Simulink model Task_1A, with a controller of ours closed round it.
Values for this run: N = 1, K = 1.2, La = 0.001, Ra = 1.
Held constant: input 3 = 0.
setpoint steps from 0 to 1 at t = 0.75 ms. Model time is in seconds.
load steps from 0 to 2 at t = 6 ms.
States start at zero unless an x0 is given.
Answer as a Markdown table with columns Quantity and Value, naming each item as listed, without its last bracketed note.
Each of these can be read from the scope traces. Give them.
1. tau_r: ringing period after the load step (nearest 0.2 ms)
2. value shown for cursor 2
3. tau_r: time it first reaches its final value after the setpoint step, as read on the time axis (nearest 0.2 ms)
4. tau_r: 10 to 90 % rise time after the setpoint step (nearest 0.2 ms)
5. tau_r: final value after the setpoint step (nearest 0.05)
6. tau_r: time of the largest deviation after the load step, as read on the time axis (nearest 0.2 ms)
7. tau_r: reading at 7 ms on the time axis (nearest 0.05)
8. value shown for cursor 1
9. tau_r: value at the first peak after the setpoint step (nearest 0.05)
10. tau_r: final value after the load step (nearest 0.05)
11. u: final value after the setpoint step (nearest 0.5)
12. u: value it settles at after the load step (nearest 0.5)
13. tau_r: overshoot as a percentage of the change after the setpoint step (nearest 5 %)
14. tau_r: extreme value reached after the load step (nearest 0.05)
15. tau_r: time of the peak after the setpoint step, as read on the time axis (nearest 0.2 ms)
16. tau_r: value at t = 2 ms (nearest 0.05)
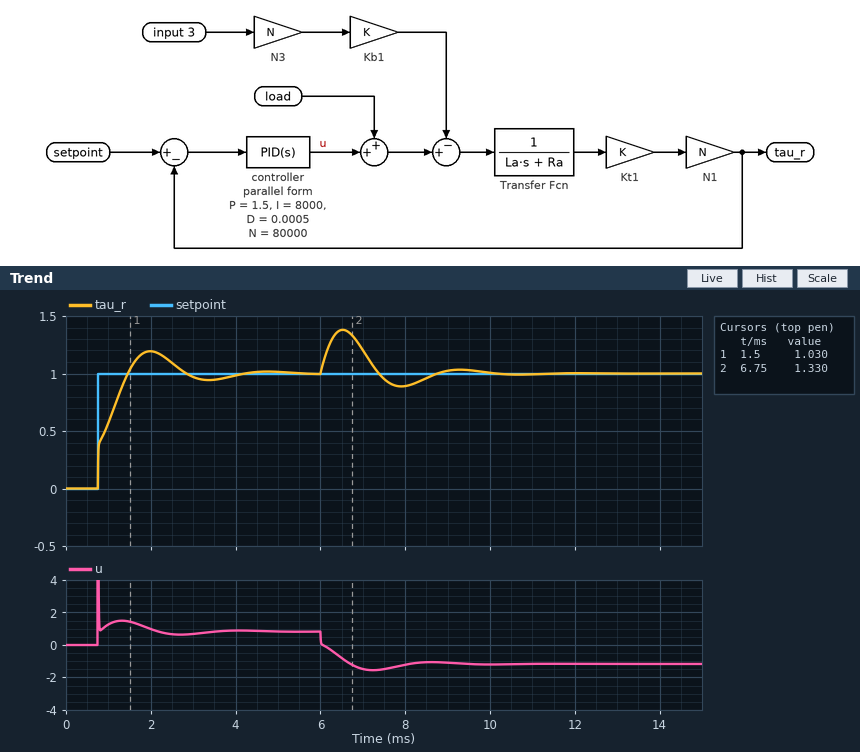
| Quantity | Value |
|---|---|
| tau_r: ringing period after the load step | 2.8 ms |
| value shown for cursor 2 | 1.330 |
| tau_r: time it first reaches its final value after the setpoint step, as read on the time axis | 1.4 ms |
| tau_r: 10 to 90 % rise time after the setpoint step | 0.6 ms |
| tau_r: final value after the setpoint step | 1.00 |
| tau_r: time of the largest deviation after the load step, as read on the time axis | 6.6 ms |
| tau_r: reading at 7 ms on the time axis | 1.20 |
| value shown for cursor 1 | 1.030 |
| tau_r: value at the first peak after the setpoint step | 1.20 |
| tau_r: final value after the load step | 1.00 |
| u: final value after the setpoint step | 1.0 |
| u: value it settles at after the load step | -1.0 |
| tau_r: overshoot as a percentage of the change after the setpoint step | 20 % |
| tau_r: extreme value reached after the load step | 1.40 |
| tau_r: time of the peak after the setpoint step, as read on the time axis | 2.0 ms |
| tau_r: value at t = 2 ms | 1.20 |
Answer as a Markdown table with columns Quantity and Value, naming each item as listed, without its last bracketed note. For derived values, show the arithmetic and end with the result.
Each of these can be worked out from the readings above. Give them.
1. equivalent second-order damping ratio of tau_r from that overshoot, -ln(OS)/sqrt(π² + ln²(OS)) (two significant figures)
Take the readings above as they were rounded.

| Quantity | Value |
|---|---|
| equivalent second-order damping ratio of tau_r from that overshoot, -ln(OS)/sqrt(π² + ln²(OS)) | ln(0.2) = -1.609; 1.609 / sqrt(9.870 + 2.590) = 0.46 |
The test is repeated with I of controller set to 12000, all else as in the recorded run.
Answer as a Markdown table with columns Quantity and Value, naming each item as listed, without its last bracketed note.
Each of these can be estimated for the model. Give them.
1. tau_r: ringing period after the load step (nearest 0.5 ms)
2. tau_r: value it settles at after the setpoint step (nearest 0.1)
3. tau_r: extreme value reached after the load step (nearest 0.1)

| Quantity | Value |
|---|---|
| tau_r: ringing period after the load step | 2.0 ms |
| tau_r: value it settles at after the setpoint step | 1.0 |
| tau_r: extreme value reached after the load step | 1.3 |
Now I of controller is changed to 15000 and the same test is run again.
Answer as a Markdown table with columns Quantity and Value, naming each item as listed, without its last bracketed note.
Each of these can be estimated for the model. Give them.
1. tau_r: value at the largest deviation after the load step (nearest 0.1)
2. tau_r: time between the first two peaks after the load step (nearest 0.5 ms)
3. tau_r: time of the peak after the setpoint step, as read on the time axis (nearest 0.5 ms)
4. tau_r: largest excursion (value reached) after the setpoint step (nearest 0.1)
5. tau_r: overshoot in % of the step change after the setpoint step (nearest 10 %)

| Quantity | Value |
|---|---|
| tau_r: value at the largest deviation after the load step | 1.3 |
| tau_r: time between the first two peaks after the load step | 2.0 ms |
| tau_r: time of the peak after the setpoint step, as read on the time axis | 1.5 ms |
| tau_r: largest excursion (value reached) after the setpoint step | 1.3 |
| tau_r: overshoot in % of the step change after the setpoint step | 30 % |
